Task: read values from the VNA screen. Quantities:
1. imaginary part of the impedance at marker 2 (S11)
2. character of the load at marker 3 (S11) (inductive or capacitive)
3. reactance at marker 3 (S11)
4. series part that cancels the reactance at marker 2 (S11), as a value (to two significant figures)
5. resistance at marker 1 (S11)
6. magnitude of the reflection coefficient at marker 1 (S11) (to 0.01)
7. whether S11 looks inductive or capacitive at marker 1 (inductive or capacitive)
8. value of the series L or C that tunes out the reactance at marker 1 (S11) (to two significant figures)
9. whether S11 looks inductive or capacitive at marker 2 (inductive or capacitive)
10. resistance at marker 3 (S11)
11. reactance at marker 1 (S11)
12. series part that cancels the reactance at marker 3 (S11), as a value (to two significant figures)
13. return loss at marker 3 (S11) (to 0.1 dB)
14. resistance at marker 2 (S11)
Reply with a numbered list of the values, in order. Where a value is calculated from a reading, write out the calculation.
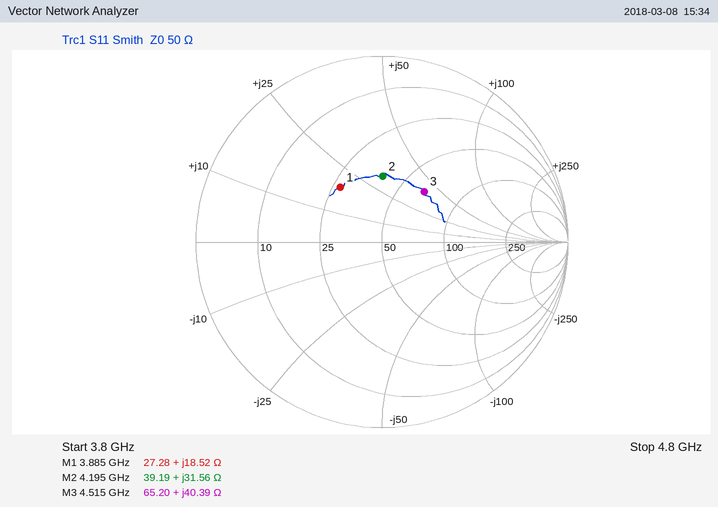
1. +31.56 Ω
2. inductive
3. +40.39 Ω
4. C = 1/(2π × 4.195 GHz × 31.56 Ω) ≈ 1.2 pF
5. 27.28 Ω
6. 0.37
7. inductive
8. C = 1/(2π × 3.885 GHz × 18.52 Ω) ≈ 2.2 pF
9. inductive
10. 65.20 Ω
11. +18.52 Ω
12. C = 1/(2π × 4.515 GHz × 40.39 Ω) ≈ 873 fF, so 870 fF to two significant figures
13. 9.0 dB
14. 39.19 Ω
